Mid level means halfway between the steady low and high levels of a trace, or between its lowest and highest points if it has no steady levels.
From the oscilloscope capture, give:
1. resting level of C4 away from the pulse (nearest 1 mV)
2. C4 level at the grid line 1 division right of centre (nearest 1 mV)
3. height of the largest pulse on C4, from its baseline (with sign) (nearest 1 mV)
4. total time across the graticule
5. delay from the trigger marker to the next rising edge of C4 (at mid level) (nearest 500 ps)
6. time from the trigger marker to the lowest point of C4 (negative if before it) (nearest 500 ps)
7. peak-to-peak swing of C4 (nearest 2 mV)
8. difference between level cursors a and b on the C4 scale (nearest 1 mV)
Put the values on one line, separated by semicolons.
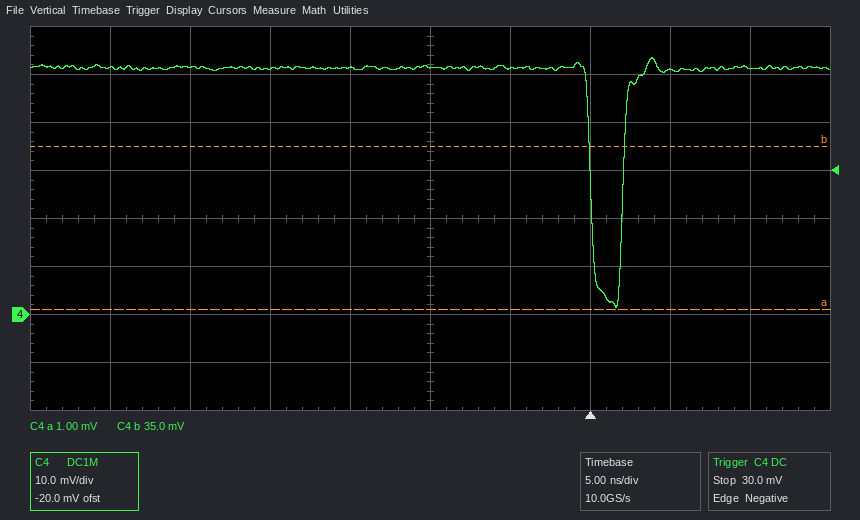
51 mV; 51 mV; -50 mV; 50 ns; 2.0 ns; +1.5 ns; 52 mV; 34 mV
